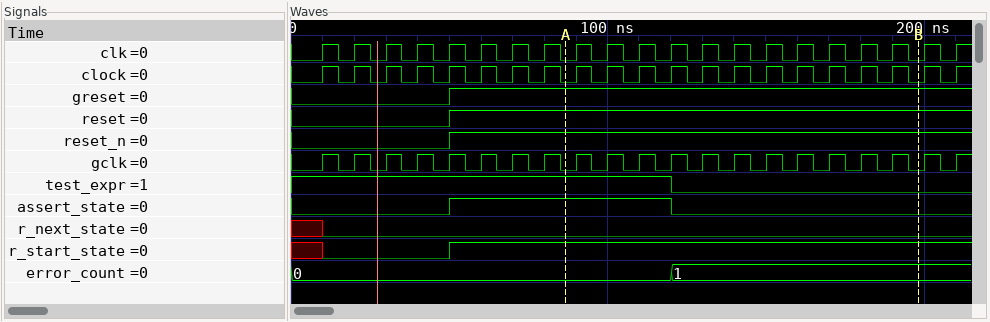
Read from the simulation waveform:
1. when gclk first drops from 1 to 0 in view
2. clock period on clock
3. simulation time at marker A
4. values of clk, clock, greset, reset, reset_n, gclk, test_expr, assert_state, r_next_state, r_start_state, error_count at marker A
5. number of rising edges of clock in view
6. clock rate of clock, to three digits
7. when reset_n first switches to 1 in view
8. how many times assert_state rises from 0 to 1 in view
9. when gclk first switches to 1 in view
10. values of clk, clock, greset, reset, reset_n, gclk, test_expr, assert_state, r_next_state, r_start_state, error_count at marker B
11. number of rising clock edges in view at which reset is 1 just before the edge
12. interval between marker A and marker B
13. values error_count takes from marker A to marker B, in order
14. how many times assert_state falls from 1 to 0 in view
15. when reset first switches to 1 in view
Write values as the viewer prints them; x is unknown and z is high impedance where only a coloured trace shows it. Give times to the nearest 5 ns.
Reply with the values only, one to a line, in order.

15 ns
10 ns
85 ns
clk=0, clock=0, greset=1, reset=1, reset_n=1, gclk=0, test_expr=1, assert_state=1, r_next_state=0, r_start_state=1, error_count=0
21
100 MHz
50 ns
1
10 ns
clk=0, clock=0, greset=1, reset=1, reset_n=1, gclk=0, test_expr=0, assert_state=0, r_next_state=0, r_start_state=1, error_count=1
16
110 ns
0, 1
1
50 ns
